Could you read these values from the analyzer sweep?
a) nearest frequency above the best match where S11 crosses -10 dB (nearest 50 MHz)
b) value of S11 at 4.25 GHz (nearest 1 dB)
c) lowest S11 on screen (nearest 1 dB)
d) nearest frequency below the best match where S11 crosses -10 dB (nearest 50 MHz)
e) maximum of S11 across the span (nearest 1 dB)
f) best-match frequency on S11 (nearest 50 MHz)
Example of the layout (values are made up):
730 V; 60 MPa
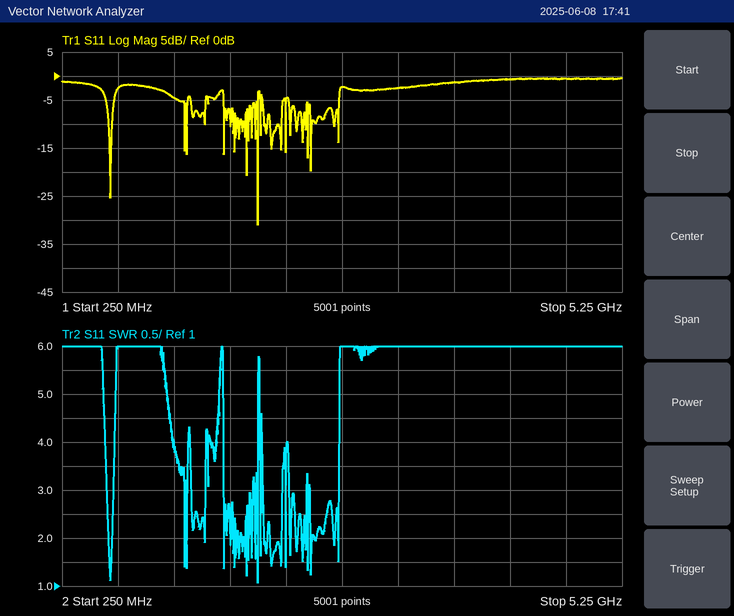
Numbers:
2.00 GHz; -1 dB; -31 dB; 2.00 GHz; 0 dB; 2.00 GHz
